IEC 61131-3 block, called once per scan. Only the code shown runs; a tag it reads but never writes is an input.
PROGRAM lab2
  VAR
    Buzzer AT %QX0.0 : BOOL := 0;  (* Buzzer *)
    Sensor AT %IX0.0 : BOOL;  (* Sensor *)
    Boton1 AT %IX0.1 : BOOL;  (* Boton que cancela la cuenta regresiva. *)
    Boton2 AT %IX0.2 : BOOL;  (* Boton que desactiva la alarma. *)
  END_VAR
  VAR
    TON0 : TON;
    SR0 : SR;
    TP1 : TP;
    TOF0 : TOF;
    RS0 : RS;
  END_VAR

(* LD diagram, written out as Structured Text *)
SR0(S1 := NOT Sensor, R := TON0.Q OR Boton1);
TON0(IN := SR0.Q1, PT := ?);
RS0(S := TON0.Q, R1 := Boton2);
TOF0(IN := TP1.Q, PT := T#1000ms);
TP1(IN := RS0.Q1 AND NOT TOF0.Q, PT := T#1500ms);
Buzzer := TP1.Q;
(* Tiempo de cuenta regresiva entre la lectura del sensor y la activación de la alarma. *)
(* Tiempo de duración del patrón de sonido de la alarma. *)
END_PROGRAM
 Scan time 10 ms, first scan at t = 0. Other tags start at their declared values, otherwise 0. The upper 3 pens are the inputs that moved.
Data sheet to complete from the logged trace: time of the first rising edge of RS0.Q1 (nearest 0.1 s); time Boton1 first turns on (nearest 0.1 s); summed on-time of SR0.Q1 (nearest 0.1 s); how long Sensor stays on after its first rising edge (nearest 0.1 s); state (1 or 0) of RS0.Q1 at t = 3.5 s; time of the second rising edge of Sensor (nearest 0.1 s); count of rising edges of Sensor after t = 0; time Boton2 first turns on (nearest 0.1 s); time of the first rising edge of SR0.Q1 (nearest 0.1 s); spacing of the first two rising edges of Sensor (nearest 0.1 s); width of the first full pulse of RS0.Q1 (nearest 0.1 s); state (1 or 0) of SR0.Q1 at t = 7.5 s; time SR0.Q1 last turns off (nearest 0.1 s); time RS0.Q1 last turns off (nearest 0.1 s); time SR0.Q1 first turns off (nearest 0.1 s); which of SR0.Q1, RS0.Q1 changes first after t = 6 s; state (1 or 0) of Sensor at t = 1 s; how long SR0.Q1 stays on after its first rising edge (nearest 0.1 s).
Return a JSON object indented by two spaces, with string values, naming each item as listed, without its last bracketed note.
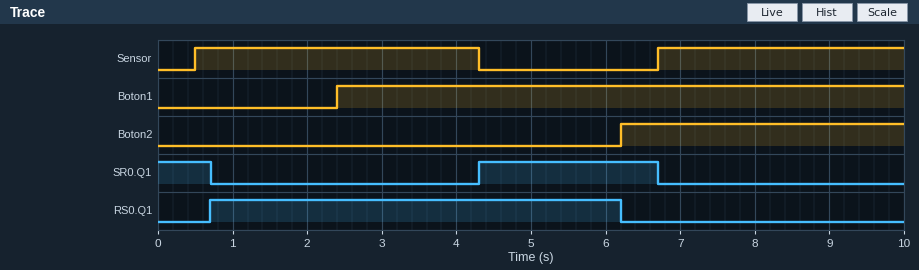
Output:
{
  "time of the first rising edge of RS0.Q1": "0.7 s",
  "time Boton1 first turns on": "2.4 s",
  "summed on-time of SR0.Q1": "3.1 s",
  "how long Sensor stays on after its first rising edge": "3.8 s",
  "state (1 or 0) of RS0.Q1 at t = 3.5 s": "1",
  "time of the second rising edge of Sensor": "6.7 s",
  "count of rising edges of Sensor after t = 0": "2",
  "time Boton2 first turns on": "6.2 s",
  "time of the first rising edge of SR0.Q1": "4.3 s",
  "spacing of the first two rising edges of Sensor": "6.2 s",
  "width of the first full pulse of RS0.Q1": "5.5 s",
  "state (1 or 0) of SR0.Q1 at t = 7.5 s": "0",
  "time SR0.Q1 last turns off": "6.7 s",
  "time RS0.Q1 last turns off": "6.2 s",
  "time SR0.Q1 first turns off": "0.7 s",
  "which of SR0.Q1, RS0.Q1 changes first after t = 6 s": "RS0.Q1",
  "state (1 or 0) of Sensor at t = 1 s": "1",
  "how long SR0.Q1 stays on after its first rising edge": "2.4 s"
}
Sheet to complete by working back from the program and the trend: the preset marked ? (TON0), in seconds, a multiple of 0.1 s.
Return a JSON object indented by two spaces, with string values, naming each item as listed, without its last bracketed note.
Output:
{
  "the preset marked ? (TON0), in seconds, a multiple of 0.1 s": "0.7 s"
}
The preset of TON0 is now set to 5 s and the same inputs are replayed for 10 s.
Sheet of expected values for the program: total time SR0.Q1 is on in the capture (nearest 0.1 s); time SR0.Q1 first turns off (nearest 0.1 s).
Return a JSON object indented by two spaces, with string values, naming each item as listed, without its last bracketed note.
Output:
{
  "total time SR0.Q1 is on in the capture": "4.8 s",
  "time SR0.Q1 first turns off": "2.4 s"
}
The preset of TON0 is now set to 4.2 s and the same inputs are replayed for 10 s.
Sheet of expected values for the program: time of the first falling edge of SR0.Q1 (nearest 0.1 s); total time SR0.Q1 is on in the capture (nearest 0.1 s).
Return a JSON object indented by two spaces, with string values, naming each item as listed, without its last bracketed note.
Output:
{
  "time of the first falling edge of SR0.Q1": "2.4 s",
  "total time SR0.Q1 is on in the capture": "4.8 s"
}
